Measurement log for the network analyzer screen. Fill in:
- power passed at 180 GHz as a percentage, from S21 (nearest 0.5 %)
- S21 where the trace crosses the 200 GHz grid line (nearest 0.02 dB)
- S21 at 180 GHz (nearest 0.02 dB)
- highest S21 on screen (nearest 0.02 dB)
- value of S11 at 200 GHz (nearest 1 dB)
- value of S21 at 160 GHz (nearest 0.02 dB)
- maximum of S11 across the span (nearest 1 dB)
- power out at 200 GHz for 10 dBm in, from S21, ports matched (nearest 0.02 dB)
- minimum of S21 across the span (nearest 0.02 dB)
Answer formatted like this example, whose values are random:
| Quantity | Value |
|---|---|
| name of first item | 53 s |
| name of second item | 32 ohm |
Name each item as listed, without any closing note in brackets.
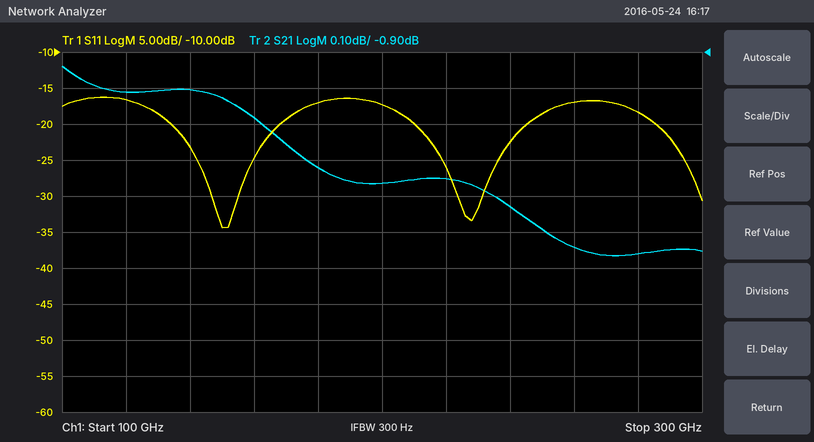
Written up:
| Quantity | Value |
|---|---|
| power passed at 180 GHz as a percentage, from S21 | 75.5 % |
| S21 where the trace crosses the 200 GHz grid line | -1.26 dB |
| S21 at 180 GHz | -1.22 dB |
| highest S21 on screen | -0.94 dB |
| value of S11 at 200 GHz | -17 dB |
| value of S21 at 160 GHz | -1.08 dB |
| maximum of S11 across the span | -16 dB |
| power out at 200 GHz for 10 dBm in, from S21, ports matched | 8.74 dBm |
| minimum of S21 across the span | -1.46 dB |
